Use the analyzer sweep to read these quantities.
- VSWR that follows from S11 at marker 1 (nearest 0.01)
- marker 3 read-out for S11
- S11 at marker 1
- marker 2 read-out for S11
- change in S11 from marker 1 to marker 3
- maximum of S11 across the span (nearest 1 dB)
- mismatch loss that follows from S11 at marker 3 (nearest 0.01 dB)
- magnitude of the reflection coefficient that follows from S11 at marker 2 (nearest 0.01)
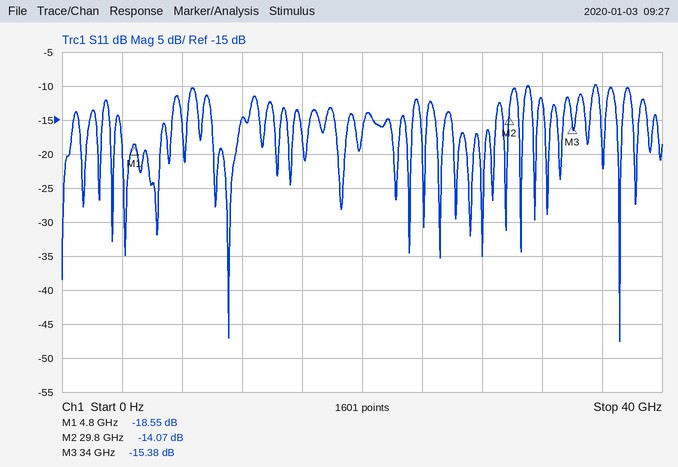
1.27
-15.38 dB
-18.55 dB
-14.07 dB
3.17 dB
-10 dB
0.13 dB
0.20
